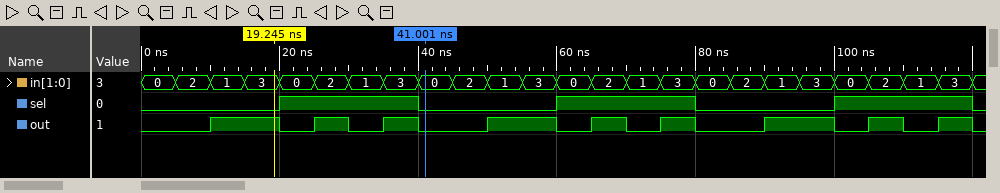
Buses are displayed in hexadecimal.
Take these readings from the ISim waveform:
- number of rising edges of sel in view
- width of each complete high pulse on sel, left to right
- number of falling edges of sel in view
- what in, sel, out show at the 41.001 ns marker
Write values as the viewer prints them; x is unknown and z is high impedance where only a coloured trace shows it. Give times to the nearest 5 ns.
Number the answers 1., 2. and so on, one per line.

1. 3
2. 20 ns, 20 ns, 20 ns
3. 3
4. in=0, sel=0, out=0
